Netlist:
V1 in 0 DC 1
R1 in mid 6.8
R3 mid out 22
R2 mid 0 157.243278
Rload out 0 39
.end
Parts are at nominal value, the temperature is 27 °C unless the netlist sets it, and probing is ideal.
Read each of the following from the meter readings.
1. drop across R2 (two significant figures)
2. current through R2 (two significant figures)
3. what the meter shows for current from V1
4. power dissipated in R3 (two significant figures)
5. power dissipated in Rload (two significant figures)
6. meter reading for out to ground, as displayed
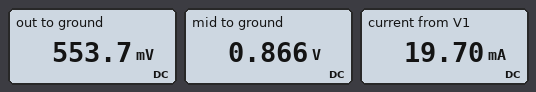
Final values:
870 mV
5.5 mA
19.70 mA
4.4 mW
7.9 mW
553.7 mV
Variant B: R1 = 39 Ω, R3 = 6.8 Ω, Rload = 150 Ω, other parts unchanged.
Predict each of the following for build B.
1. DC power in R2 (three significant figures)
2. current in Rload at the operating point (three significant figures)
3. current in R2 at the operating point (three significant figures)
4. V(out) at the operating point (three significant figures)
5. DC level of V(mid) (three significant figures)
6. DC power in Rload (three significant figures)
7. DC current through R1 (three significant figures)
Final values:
2.84 mW
4.26 mA
4.25 mA
639 mV
668 mV
2.72 mW
8.51 mA
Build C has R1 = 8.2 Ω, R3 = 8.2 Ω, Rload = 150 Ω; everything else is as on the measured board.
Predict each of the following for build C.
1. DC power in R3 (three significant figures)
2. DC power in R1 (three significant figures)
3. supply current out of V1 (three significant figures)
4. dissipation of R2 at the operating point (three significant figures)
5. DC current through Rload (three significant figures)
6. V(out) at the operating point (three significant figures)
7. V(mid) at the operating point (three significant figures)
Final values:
269 µW
1.08 mW
11.5 mA
5.22 mW
5.73 mA
859 mV
906 mV
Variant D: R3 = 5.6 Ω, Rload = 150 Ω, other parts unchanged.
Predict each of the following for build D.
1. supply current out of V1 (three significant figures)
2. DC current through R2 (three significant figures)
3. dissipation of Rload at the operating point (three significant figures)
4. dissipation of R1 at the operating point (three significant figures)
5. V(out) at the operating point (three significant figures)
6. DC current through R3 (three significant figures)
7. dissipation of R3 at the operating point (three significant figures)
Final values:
11.8 mA
5.85 mA
5.24 mW
941 µW
887 mV
5.91 mA
196 µW
